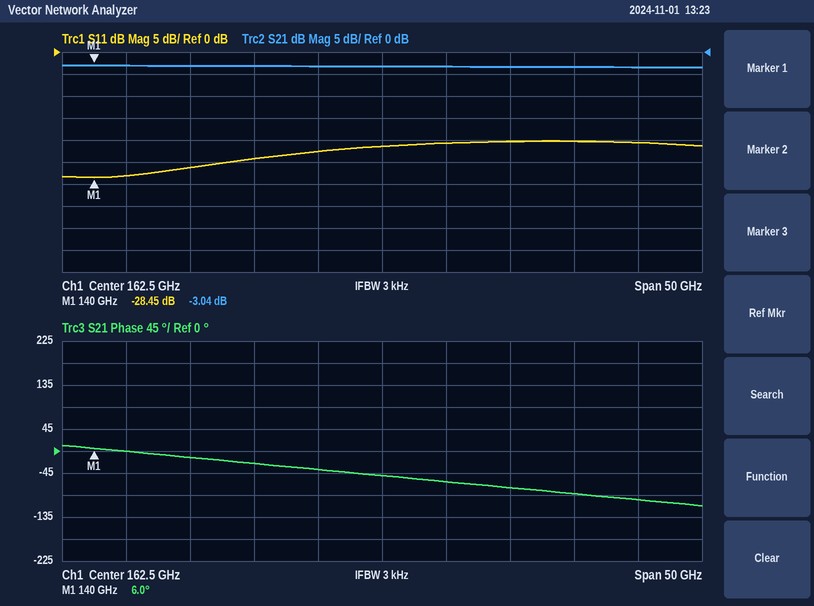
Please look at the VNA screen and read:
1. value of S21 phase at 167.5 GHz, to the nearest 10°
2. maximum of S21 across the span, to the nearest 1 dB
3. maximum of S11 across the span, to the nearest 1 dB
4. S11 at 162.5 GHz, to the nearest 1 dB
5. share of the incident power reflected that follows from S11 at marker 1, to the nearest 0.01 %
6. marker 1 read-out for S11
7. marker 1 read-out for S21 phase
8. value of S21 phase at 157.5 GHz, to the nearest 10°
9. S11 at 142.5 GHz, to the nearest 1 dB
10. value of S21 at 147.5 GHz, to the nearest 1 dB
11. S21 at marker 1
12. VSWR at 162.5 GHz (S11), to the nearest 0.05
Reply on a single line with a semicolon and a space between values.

-60°; -3 dB; -20 dB; -21 dB; 0.14 %; -28.45 dB; 6.0°; -40°; -28 dB; -3 dB; -3.04 dB; 1.20
